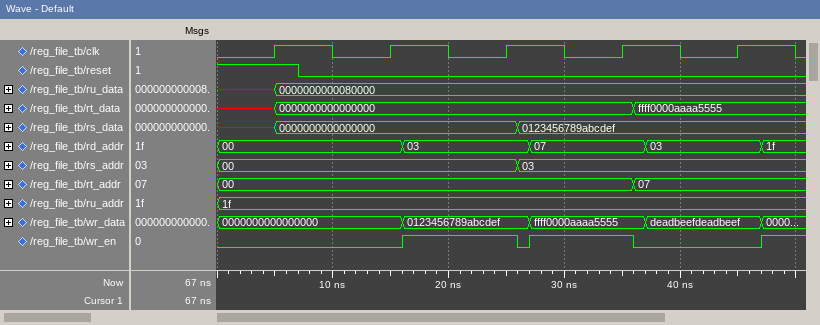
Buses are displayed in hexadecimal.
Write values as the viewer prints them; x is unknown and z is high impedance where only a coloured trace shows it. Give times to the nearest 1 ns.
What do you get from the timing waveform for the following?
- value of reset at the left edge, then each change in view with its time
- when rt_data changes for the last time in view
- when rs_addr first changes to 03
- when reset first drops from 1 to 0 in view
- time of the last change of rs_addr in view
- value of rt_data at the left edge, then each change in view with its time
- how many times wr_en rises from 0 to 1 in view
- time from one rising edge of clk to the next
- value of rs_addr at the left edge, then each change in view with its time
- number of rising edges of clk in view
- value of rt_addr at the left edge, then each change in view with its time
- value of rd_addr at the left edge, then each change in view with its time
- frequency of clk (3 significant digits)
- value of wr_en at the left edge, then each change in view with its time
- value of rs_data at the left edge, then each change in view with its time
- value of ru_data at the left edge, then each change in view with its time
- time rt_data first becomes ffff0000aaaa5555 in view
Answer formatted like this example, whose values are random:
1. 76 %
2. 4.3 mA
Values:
1. 1, 0 at 7 ns
2. 36 ns
3. 26 ns
4. 7 ns
5. 26 ns
6. x, 0000000000000000 at 5 ns, ffff0000aaaa5555 at 36 ns
7. 3
8. 10 ns
9. 00, 03 at 26 ns
10. 5
11. 00, 07 at 36 ns
12. 00, 03 at 16 ns, 07 at 27 ns, 03 at 37 ns, 1f at 47 ns
13. 100 MHz
14. 0, 1 at 16 ns, 0 at 26 ns, 1 at 27 ns, 0 at 36 ns, 1 at 47 ns
15. x, 0000000000000000 at 5 ns, 0123456789abcdef at 26 ns
16. x, 0000000000080000 at 5 ns
17. 36 ns
